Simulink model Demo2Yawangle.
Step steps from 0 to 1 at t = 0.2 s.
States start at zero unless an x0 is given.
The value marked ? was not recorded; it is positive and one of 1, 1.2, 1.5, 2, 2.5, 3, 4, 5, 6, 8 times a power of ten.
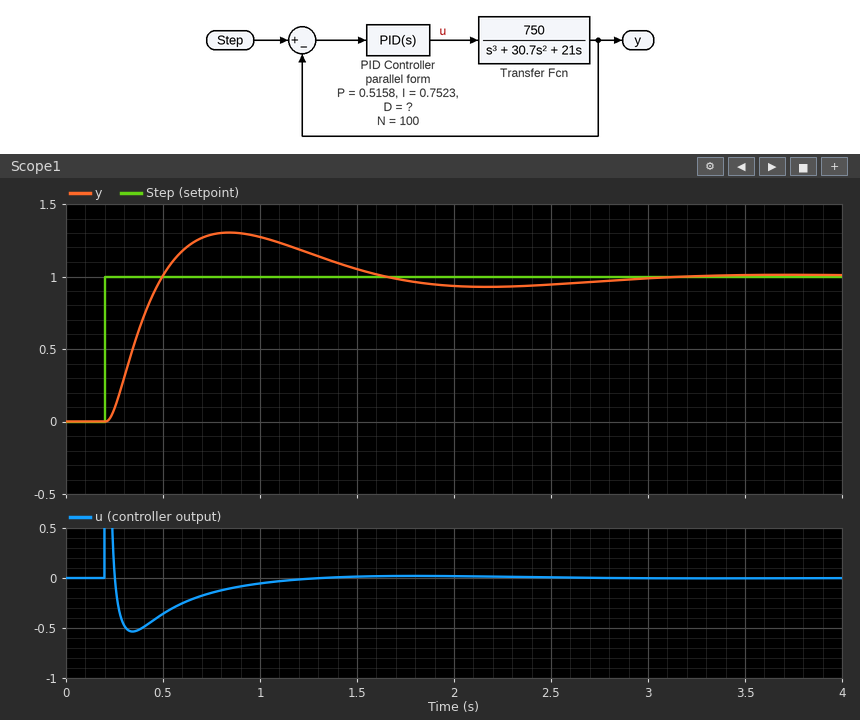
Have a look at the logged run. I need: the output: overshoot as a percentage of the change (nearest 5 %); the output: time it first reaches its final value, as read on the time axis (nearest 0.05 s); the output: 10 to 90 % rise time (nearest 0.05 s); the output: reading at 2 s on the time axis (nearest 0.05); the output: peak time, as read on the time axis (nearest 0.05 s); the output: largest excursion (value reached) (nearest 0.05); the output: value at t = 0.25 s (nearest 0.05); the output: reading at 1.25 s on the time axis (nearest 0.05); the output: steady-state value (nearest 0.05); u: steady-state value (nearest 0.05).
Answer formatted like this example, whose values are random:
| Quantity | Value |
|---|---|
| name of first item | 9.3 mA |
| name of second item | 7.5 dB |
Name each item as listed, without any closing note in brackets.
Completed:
| Quantity | Value |
|---|---|
| the output: overshoot as a percentage of the change | 30 % |
| the output: time it first reaches its final value, as read on the time axis | 0.50 s |
| the output: 10 to 90 % rise time | 0.20 s |
| the output: reading at 2 s on the time axis | 0.95 |
| the output: peak time, as read on the time axis | 0.85 s |
| the output: largest excursion (value reached) | 1.30 |
| the output: value at t = 0.25 s | 0.10 |
| the output: reading at 1.25 s on the time axis | 1.15 |
| the output: steady-state value | 1.00 |
| u: steady-state value | 0.00 |
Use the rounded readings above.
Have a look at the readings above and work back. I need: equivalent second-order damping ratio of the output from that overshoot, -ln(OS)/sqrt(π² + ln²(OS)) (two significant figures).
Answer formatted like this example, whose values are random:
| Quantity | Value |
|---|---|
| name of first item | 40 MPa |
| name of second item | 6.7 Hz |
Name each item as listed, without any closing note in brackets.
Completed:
| Quantity | Value |
|---|---|
| equivalent second-order damping ratio of the output from that overshoot, -ln(OS)/sqrt(π² + ln²(OS)) | 0.36 |
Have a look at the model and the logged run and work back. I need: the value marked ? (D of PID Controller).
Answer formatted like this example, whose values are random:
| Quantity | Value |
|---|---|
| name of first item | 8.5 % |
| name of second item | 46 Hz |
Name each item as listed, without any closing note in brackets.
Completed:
| Quantity | Value |
|---|---|
| the value marked ? | 0.2 |
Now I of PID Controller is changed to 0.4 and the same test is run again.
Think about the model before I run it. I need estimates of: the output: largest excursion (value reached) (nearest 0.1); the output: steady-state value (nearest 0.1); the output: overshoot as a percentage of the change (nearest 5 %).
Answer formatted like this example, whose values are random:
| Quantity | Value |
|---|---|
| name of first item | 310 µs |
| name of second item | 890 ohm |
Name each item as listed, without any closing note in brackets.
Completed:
| Quantity | Value |
|---|---|
| the output: largest excursion (value reached) | 1.2 |
| the output: steady-state value | 1.0 |
| the output: overshoot as a percentage of the change | 25 % |
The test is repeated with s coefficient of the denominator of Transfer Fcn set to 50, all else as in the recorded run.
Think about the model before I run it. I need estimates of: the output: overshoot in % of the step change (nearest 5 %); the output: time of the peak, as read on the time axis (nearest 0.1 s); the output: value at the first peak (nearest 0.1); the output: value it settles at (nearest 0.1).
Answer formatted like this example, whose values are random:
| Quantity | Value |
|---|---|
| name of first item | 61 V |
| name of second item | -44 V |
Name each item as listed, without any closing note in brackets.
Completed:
| Quantity | Value |
|---|---|
| the output: overshoot in % of the step change | 20 % |
| the output: time of the peak, as read on the time axis | 1.0 s |
| the output: value at the first peak | 1.2 |
| the output: value it settles at | 1.0 |
